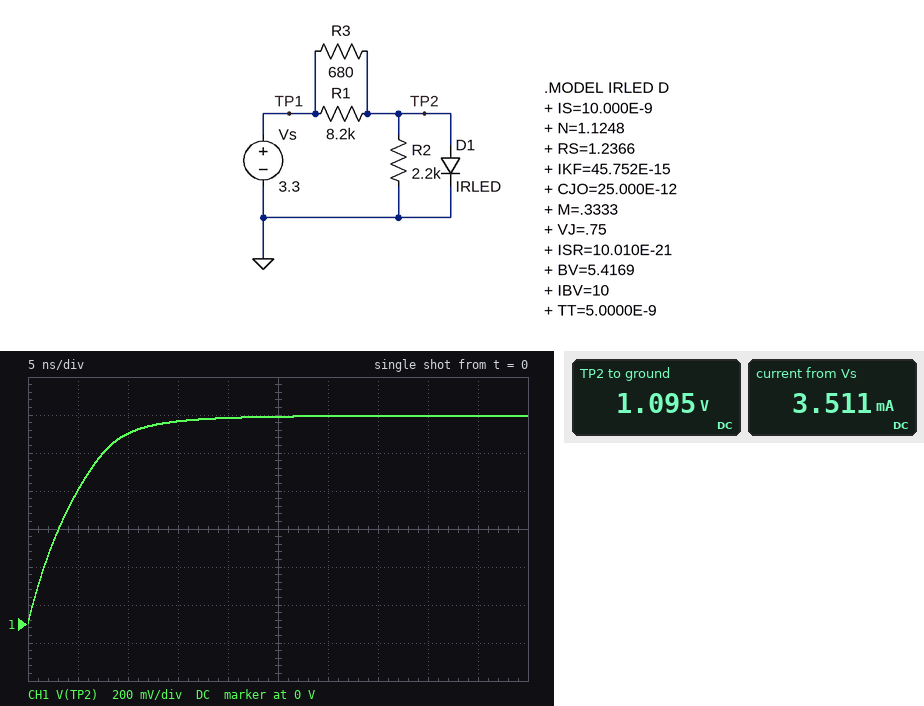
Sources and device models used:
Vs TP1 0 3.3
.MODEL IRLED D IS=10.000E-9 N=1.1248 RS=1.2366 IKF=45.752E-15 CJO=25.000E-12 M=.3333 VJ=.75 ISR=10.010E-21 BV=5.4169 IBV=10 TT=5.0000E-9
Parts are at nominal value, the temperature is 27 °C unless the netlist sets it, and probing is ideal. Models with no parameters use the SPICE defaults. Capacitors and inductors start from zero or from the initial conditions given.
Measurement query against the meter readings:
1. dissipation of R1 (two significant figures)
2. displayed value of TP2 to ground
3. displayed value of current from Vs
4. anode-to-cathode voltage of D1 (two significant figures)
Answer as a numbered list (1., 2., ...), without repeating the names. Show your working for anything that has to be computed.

1. (3.3 V - 1.095 V)^2 / 8.2 kΩ = 590 µW
2. 1.095 V
3. 3.511 mA
4. 1.095 V = 1.1 V
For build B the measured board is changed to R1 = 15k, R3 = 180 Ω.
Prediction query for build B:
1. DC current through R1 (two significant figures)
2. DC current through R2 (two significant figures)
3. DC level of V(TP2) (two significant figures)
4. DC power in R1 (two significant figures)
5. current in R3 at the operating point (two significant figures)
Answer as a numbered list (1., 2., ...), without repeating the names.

1. 140 µA
2. 540 µA
3. 1.2 V
4. 300 µW
5. 12 mA
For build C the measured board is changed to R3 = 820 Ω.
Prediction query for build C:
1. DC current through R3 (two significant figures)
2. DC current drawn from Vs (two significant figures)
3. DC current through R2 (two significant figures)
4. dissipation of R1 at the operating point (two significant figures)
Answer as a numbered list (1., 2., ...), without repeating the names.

1. 2.7 mA
2. 3.0 mA
3. 490 µA
4. 600 µW
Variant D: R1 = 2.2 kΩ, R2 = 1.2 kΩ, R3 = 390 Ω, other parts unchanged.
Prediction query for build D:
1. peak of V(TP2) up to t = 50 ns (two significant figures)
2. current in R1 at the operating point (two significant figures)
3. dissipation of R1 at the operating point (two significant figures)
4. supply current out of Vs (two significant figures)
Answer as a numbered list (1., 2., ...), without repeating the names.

1. 1.1 V
2. 980 µA
3. 2.1 mW
4. 6.5 mA
